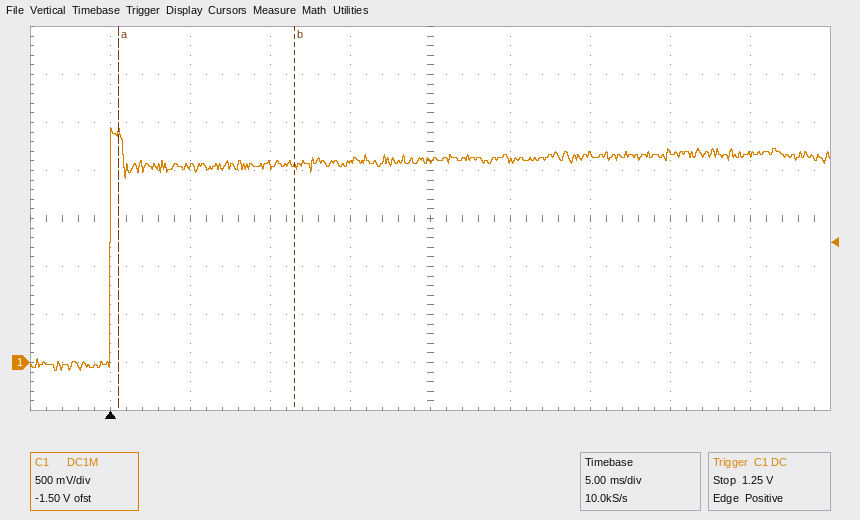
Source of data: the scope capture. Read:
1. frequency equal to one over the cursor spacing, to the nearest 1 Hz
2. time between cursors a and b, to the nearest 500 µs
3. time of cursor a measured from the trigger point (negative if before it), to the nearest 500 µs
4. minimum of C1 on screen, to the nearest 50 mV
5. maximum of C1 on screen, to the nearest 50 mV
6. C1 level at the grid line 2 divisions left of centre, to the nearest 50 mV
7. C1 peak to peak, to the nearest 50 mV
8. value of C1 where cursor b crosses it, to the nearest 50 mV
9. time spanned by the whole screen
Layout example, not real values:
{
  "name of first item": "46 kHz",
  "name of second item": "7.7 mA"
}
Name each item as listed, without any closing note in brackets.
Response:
{
  "frequency equal to one over the cursor spacing, to the nearest 1 Hz": "91 Hz",
  "time between cursors a and b, to the nearest 500 µs": "11.0 ms",
  "time of cursor a measured from the trigger point (negative if before it), to the nearest 500 µs": "+500 µs",
  "minimum of C1 on screen, to the nearest 50 mV": "-100 mV",
  "maximum of C1 on screen, to the nearest 50 mV": "2.45 V",
  "C1 level at the grid line 2 divisions left of centre, to the nearest 50 mV": "2.05 V",
  "C1 peak to peak, to the nearest 50 mV": "2.55 V",
  "value of C1 where cursor b crosses it, to the nearest 50 mV": "2.05 V",
  "time spanned by the whole screen": "50 ms"
}
